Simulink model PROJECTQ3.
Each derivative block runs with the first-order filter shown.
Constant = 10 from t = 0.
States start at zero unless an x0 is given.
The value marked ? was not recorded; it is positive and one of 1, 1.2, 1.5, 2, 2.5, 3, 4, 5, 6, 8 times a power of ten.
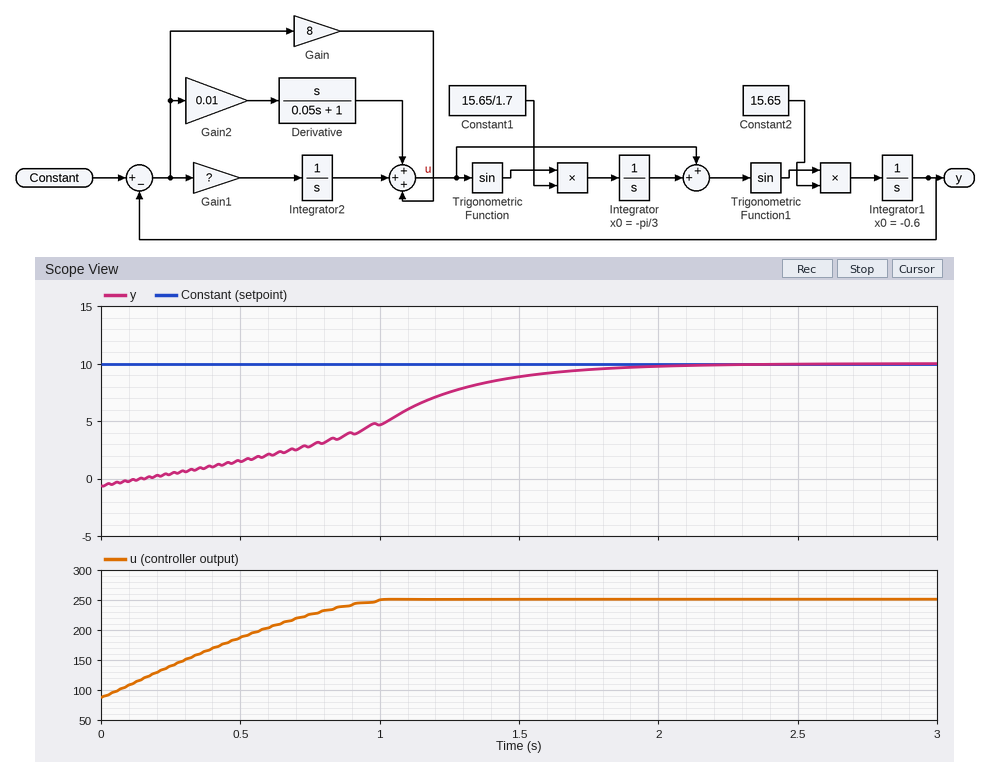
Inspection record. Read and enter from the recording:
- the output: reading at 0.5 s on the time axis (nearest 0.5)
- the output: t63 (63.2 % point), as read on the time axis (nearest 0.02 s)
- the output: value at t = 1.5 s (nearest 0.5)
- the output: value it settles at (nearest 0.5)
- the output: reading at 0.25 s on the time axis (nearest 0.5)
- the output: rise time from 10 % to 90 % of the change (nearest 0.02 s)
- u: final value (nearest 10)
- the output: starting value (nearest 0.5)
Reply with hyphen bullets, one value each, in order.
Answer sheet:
- 1.5
- 1.10 s
- 9.0
- 10.0
- 0.5
- 1.28 s
- 250
- -0.5
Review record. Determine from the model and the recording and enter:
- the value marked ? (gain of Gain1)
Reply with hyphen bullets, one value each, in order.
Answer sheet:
- 25
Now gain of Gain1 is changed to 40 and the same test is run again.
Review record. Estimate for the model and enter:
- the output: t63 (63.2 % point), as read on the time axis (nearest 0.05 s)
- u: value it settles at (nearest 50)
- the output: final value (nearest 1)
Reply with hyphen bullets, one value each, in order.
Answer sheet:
- 1.95 s
- 650
- 10
